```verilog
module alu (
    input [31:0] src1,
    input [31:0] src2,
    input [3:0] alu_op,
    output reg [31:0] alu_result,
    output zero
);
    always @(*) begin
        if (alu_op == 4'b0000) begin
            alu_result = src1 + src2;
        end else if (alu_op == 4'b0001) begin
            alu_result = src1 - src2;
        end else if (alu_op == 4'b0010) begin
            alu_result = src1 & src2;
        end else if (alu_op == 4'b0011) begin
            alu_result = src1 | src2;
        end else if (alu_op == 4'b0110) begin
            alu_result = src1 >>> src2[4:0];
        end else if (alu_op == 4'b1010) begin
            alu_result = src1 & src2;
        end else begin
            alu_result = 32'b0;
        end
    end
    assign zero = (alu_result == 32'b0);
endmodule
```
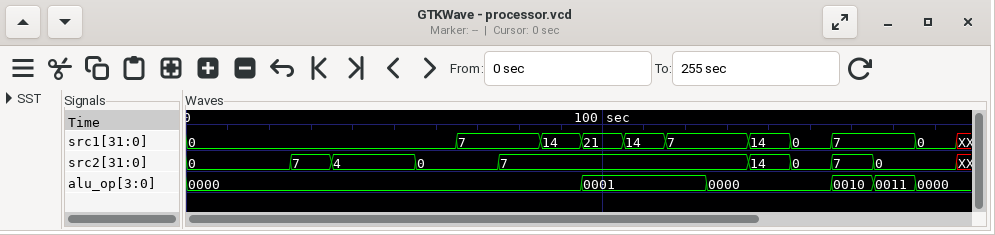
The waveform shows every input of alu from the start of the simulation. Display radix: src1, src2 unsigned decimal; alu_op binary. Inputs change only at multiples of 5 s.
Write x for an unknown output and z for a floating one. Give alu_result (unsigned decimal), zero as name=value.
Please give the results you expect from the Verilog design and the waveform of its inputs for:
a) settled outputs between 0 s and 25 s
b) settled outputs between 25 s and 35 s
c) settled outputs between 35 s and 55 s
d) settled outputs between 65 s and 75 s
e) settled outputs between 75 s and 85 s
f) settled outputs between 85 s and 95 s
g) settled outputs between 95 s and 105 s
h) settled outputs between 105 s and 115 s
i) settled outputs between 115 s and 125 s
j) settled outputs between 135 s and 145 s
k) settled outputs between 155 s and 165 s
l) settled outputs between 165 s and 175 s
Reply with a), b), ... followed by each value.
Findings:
a) alu_result=0, zero=1
b) alu_result=7, zero=0
c) alu_result=4, zero=0
d) alu_result=7, zero=0
e) alu_result=14, zero=0
f) alu_result=21, zero=0
g) alu_result=14, zero=0
h) alu_result=7, zero=0
i) alu_result=0, zero=1
j) alu_result=28, zero=0
k) alu_result=7, zero=0
l) alu_result=7, zero=0
